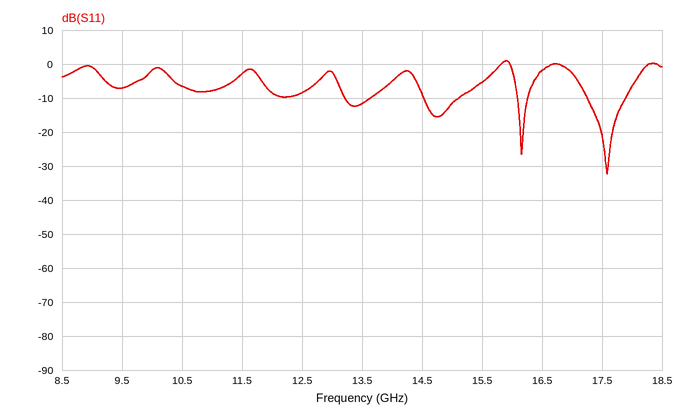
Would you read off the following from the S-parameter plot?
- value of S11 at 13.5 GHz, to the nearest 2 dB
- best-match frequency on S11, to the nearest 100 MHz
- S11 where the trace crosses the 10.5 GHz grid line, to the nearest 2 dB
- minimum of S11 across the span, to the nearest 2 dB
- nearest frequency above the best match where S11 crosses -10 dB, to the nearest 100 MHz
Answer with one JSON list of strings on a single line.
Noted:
["-12 dB", "17.6 GHz", "-6 dB", "-32 dB", "17.9 GHz"]
